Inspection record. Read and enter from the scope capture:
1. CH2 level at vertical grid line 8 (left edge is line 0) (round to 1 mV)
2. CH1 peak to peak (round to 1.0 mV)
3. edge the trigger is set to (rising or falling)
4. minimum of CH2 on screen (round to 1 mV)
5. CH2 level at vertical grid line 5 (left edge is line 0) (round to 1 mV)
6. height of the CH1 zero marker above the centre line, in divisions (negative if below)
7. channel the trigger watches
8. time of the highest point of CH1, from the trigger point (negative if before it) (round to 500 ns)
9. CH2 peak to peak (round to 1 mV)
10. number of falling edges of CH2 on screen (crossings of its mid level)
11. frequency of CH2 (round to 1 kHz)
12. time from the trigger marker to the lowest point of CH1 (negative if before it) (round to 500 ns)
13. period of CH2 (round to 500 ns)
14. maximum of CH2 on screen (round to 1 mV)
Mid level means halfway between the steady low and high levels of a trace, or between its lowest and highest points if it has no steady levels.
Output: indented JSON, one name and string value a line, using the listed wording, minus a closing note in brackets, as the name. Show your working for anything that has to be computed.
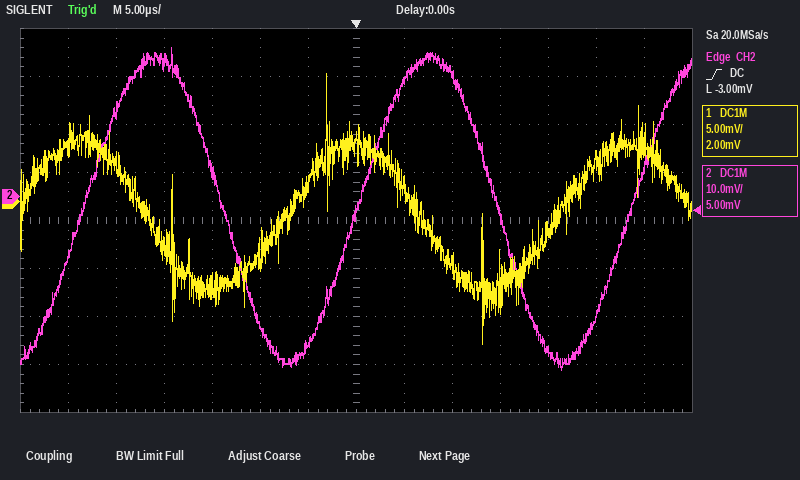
{
  "CH2 level at vertical grid line 8 (left edge is line 0)": "24 mV",
  "CH1 peak to peak": "28.0 mV",
  "edge the trigger is set to": "rising",
  "minimum of CH2 on screen": "-36 mV",
  "CH2 level at vertical grid line 5 (left edge is line 0)": "-27 mV",
  "height of the CH1 zero marker above the centre line, in divisions": "+0.4 div",
  "channel the trigger watches": "CH2",
  "time of the highest point of CH1, from the trigger point (negative if before it)": "-3.0 µs",
  "CH2 peak to peak": "31 mV − (-36 mV) = 67 mV",
  "number of falling edges of CH2 on screen": "2",
  "frequency of CH2": "1 / 28.5 µs ≈ 35 kHz",
  "time from the trigger marker to the lowest point of CH1 (negative if before it)": "+13.0 µs",
  "period of CH2": "28.5 µs",
  "maximum of CH2 on screen": "31 mV"
}
